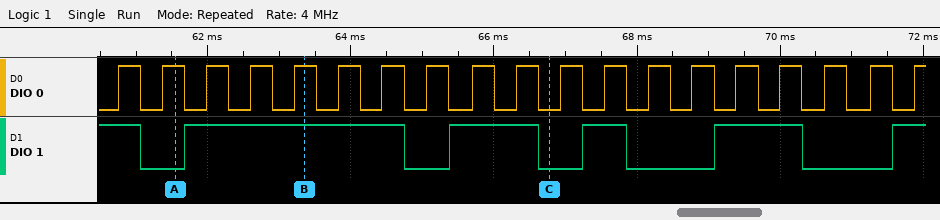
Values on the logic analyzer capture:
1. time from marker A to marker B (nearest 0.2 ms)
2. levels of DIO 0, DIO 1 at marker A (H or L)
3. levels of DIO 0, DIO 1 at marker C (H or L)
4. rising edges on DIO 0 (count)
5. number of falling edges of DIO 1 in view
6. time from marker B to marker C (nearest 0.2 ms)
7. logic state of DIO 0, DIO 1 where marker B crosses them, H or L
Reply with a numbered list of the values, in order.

1. 1.8 ms
2. DIO 0=H, DIO 1=L
3. DIO 0=L, DIO 1=L
4. 19
5. 5
6. 3.4 ms
7. DIO 0=H, DIO 1=H
